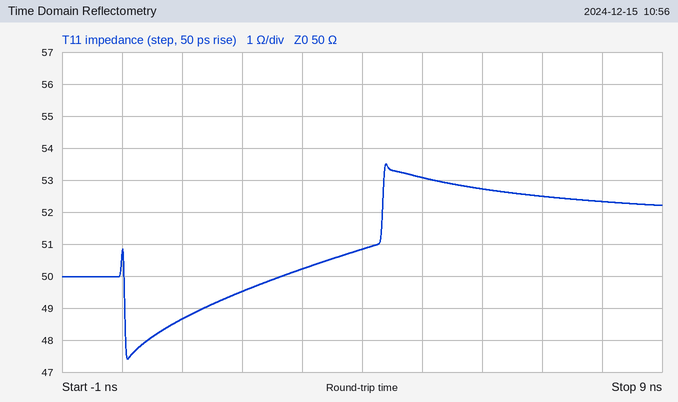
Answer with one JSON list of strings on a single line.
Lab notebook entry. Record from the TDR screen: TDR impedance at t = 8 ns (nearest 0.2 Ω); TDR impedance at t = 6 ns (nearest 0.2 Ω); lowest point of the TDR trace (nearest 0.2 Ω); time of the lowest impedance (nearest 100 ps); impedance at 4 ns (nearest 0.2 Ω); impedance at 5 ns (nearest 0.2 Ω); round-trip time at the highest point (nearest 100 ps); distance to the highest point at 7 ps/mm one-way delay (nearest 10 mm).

["52.4 Ω", "52.8 Ω", "47.4 Ω", "100 ps", "50.8 Ω", "53.0 Ω", "4.4 ns", "310 mm"]
